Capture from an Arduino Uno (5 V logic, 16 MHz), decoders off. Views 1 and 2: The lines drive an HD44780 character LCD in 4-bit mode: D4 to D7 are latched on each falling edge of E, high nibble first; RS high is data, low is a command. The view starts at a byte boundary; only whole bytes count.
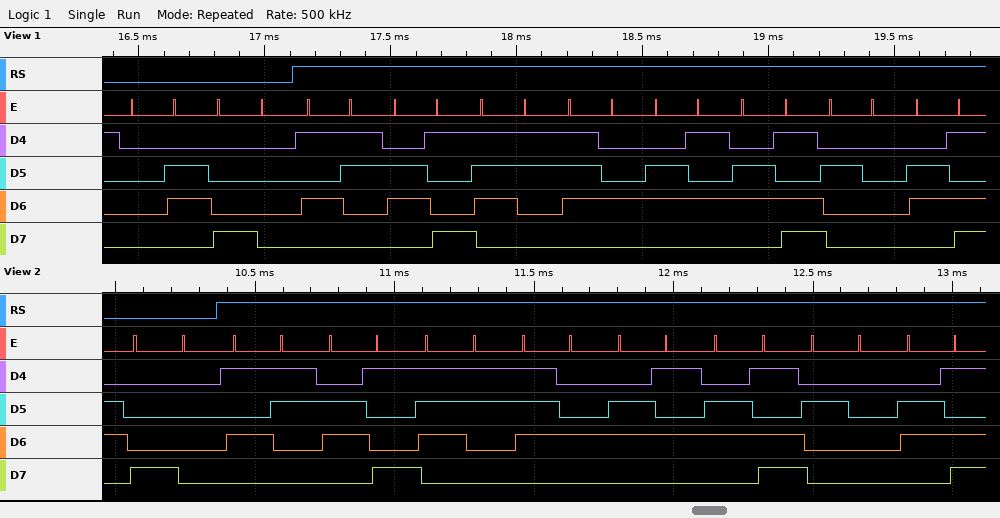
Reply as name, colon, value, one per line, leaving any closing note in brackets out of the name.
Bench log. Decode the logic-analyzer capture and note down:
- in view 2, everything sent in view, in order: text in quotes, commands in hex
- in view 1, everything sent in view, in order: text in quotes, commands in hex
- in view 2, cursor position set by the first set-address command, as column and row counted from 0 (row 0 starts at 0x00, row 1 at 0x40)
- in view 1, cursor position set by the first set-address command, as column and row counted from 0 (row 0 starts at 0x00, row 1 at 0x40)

in view 2, everything sent in view, in order: text in quotes, commands in hex: 0x80 "Sistem m"
in view 1, everything sent in view, in order: text in quotes, commands in hex: 0x06 0x80 "Sistem m"
in view 2, cursor position set by the first set-address command, as column and row counted from 0: column 0, row 0
in view 1, cursor position set by the first set-address command, as column and row counted from 0: column 0, row 0
